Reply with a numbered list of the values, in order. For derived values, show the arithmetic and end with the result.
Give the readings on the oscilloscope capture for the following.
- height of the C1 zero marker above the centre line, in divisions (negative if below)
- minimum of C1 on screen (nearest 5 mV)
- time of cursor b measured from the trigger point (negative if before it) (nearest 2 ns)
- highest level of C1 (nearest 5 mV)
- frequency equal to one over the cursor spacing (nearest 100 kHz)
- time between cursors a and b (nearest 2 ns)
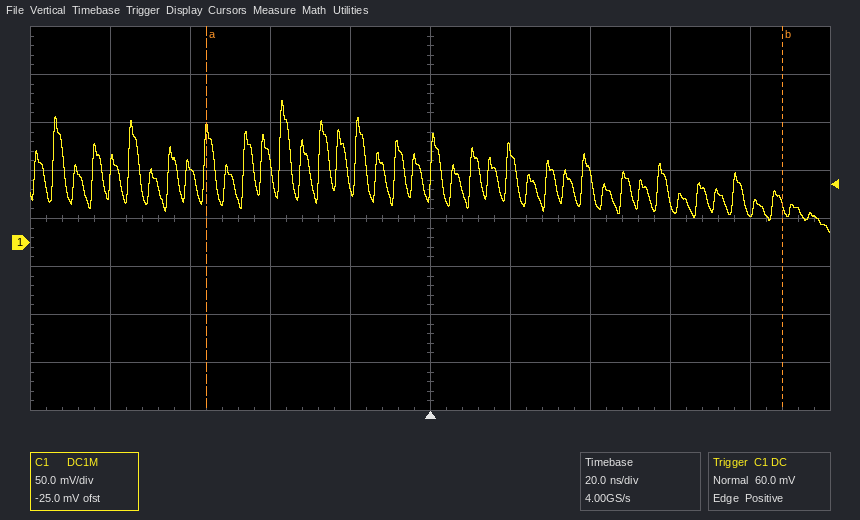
1. -0.5 div
2. 10 mV
3. +88 ns
4. 150 mV
5. 1 / 144 ns ≈ 6.9 MHz
6. 144 ns
